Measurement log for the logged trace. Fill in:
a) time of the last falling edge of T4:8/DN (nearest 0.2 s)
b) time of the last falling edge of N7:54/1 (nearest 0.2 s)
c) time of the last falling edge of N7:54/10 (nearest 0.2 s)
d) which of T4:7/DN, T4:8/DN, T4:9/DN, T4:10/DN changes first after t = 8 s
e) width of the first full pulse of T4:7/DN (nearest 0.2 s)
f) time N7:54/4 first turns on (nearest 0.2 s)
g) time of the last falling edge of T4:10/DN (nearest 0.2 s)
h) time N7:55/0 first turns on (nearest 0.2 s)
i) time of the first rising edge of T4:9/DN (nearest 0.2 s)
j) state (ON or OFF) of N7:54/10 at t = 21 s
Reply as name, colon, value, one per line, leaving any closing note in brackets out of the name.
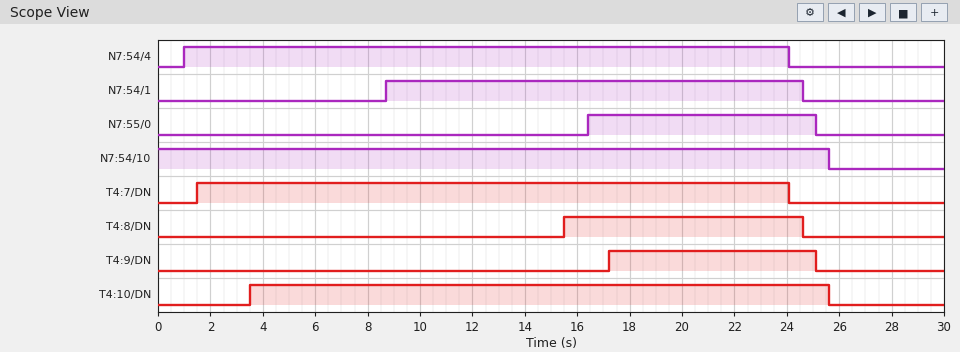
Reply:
time of the last falling edge of T4:8/DN: 24.6 s
time of the last falling edge of N7:54/1: 24.6 s
time of the last falling edge of N7:54/10: 25.6 s
which of T4:7/DN, T4:8/DN, T4:9/DN, T4:10/DN changes first after t = 8 s: T4:8/DN
width of the first full pulse of T4:7/DN: 22.6 s
time N7:54/4 first turns on: 1.0 s
time of the last falling edge of T4:10/DN: 25.6 s
time N7:55/0 first turns on: 16.4 s
time of the first rising edge of T4:9/DN: 17.2 s
state (ON or OFF) of N7:54/10 at t = 21 s: ON
